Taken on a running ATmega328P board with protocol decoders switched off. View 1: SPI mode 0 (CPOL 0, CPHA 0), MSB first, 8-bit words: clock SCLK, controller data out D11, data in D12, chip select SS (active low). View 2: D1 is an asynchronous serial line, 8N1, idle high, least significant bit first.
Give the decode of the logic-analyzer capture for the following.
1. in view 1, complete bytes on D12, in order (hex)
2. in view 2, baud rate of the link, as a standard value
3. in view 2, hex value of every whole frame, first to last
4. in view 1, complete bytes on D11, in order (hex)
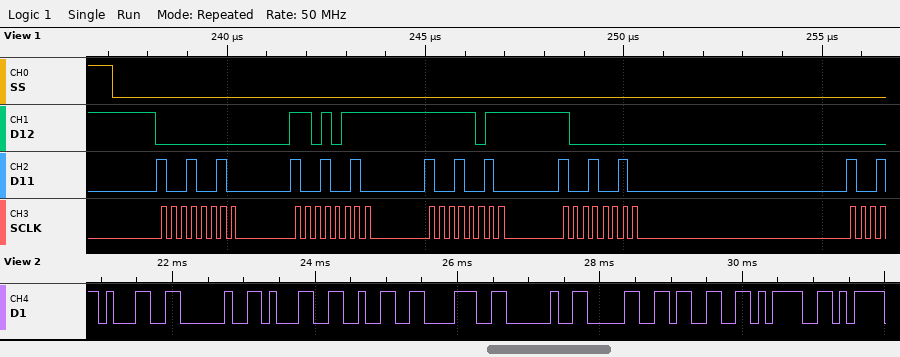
00 D7 FB 80
9600 baud
31 20 31 32 38 20 30 33 3D
92 92 92 92
